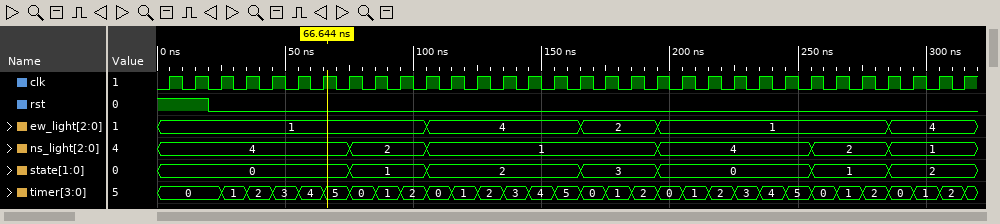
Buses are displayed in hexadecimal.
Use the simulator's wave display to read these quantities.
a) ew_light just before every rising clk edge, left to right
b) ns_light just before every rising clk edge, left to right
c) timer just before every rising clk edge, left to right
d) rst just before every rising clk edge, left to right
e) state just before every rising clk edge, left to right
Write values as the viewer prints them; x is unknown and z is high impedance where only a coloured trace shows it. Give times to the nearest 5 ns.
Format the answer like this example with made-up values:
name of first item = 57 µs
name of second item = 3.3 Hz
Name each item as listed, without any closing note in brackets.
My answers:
ew_light just before every rising clk edge, left to right = 1, 1, 1, 1, 1, 1, 1, 1, 1, 1, 1, 4, 4, 4, 4, 4, 4, 2, 2, 2, 1, 1, 1, 1, 1, 1, 1, 1, 1, 4, 4, 4
ns_light just before every rising clk edge, left to right = 4, 4, 4, 4, 4, 4, 4, 4, 2, 2, 2, 1, 1, 1, 1, 1, 1, 1, 1, 1, 4, 4, 4, 4, 4, 4, 2, 2, 2, 1, 1, 1
timer just before every rising clk edge, left to right = 0, 0, 0, 1, 2, 3, 4, 5, 0, 1, 2, 0, 1, 2, 3, 4, 5, 0, 1, 2, 0, 1, 2, 3, 4, 5, 0, 1, 2, 0, 1, 2
rst just before every rising clk edge, left to right = 1 1 0 0 0 0 0 0 0 0 0 0 0 0 0 0 0 0 0 0 0 0 0 0 0 0 0 0 0 0 0 0
state just before every rising clk edge, left to right = 0, 0, 0, 0, 0, 0, 0, 0, 1, 1, 1, 2, 2, 2, 2, 2, 2, 3, 3, 3, 0, 0, 0, 0, 0, 0, 1, 1, 1, 2, 2, 2
